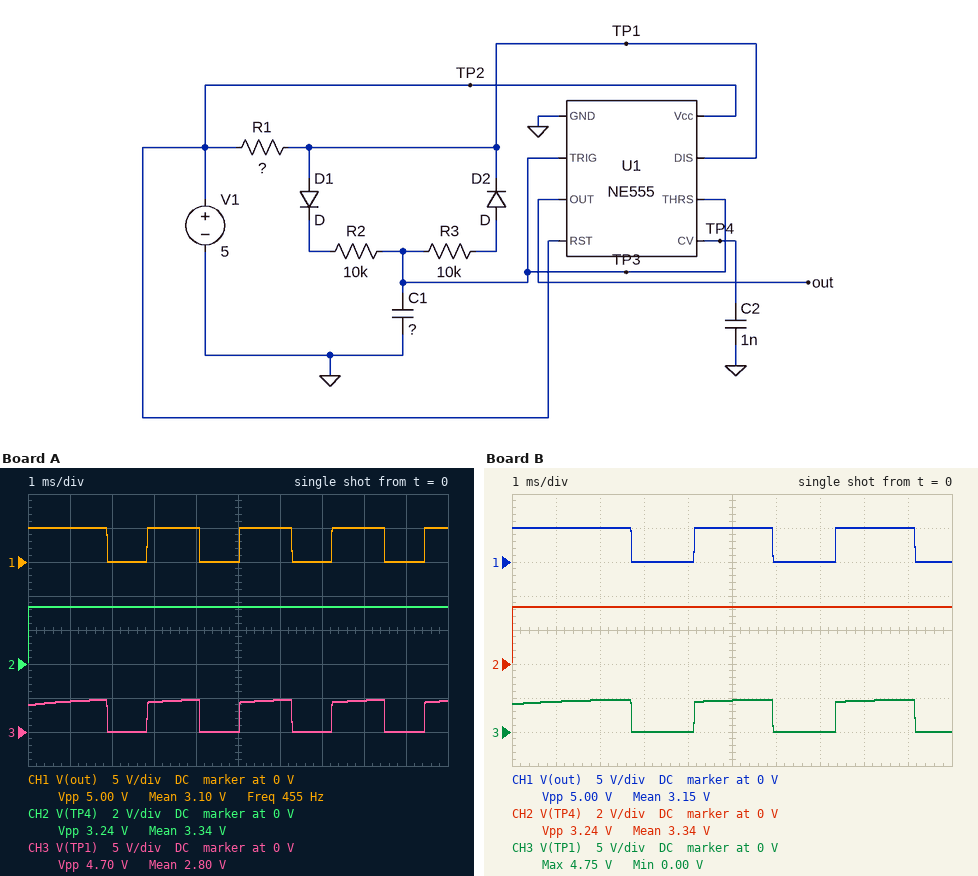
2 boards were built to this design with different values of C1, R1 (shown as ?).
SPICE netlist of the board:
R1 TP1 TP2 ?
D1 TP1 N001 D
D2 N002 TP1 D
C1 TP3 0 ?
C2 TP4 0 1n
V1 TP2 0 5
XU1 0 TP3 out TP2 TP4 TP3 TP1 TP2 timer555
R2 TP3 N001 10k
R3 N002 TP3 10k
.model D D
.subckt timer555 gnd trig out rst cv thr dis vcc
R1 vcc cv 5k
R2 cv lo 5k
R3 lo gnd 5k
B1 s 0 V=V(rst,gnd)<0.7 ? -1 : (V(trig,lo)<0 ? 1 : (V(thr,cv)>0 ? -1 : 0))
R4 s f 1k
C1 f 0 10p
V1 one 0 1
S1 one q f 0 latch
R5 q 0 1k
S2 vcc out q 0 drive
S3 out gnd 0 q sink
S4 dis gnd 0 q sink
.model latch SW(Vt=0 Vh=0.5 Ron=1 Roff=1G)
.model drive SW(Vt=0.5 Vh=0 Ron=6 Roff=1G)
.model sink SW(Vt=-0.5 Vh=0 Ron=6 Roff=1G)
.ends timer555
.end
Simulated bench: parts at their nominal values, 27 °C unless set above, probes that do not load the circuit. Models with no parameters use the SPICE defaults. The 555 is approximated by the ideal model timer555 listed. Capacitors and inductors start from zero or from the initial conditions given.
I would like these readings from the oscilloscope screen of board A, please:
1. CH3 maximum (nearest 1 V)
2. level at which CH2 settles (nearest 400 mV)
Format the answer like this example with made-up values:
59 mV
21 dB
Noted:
5 V
3.2 V
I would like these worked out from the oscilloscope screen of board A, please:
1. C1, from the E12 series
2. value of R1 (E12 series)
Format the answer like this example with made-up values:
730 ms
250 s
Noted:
100 nF
3.3 kΩ
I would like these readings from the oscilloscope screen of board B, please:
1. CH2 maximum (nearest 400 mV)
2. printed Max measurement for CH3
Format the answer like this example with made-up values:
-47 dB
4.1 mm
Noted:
3.2 V
4.75 V
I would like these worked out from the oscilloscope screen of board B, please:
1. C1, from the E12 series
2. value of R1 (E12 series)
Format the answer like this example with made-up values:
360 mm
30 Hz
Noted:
150 nF
2.7 kΩ
